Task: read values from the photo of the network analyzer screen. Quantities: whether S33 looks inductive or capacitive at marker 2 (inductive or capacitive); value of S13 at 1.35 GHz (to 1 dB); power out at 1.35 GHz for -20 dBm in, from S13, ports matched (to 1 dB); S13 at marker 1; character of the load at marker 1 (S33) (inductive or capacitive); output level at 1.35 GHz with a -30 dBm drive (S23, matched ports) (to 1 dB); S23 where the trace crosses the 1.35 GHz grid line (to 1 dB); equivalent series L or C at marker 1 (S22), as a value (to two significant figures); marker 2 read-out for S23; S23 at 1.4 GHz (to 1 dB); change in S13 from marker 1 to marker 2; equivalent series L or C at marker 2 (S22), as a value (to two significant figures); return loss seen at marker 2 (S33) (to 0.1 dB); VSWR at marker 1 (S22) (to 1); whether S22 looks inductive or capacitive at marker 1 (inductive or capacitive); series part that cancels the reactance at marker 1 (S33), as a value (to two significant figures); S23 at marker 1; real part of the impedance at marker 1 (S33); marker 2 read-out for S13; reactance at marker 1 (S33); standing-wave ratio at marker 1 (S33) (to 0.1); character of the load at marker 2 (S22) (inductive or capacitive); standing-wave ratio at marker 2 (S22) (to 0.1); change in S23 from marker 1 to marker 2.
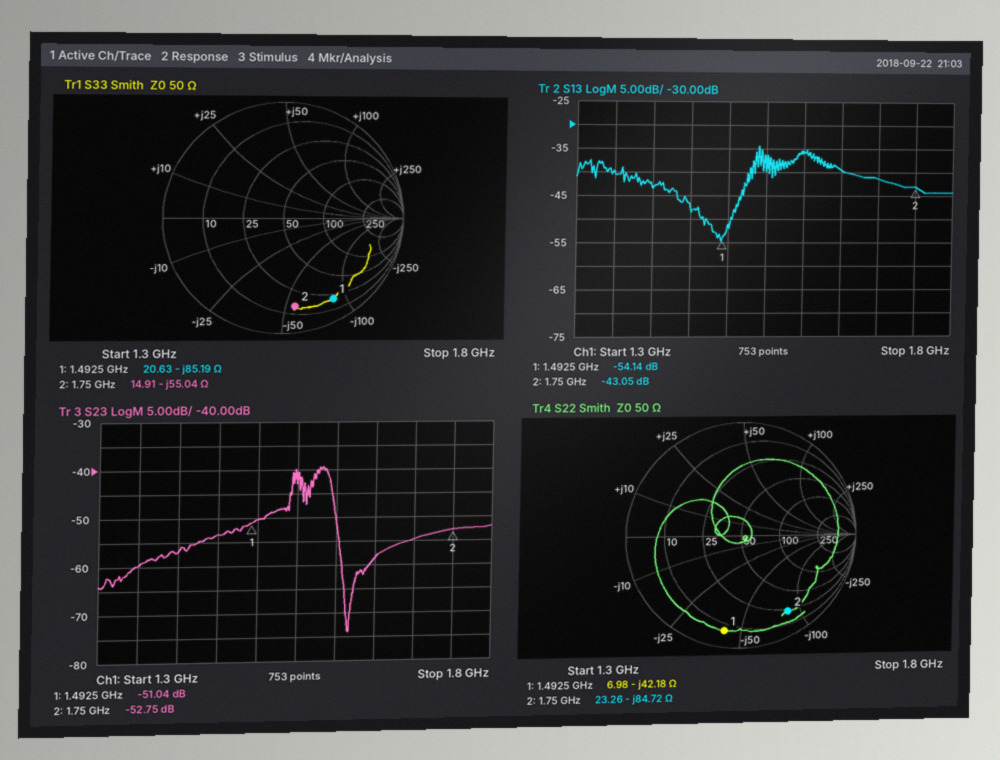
capacitive
-40 dB
-60 dBm
-54.14 dB
capacitive
-90 dBm
-60 dB
2.5 pF
-52.75 dB
-57 dB
11.09 dB
1.1 pF
2.3 dB
12
capacitive
9.1 nH
-51.04 dB
20.63 Ω
-43.05 dB
-85.19 Ω
9.8
capacitive
8.7
-1.71 dB
